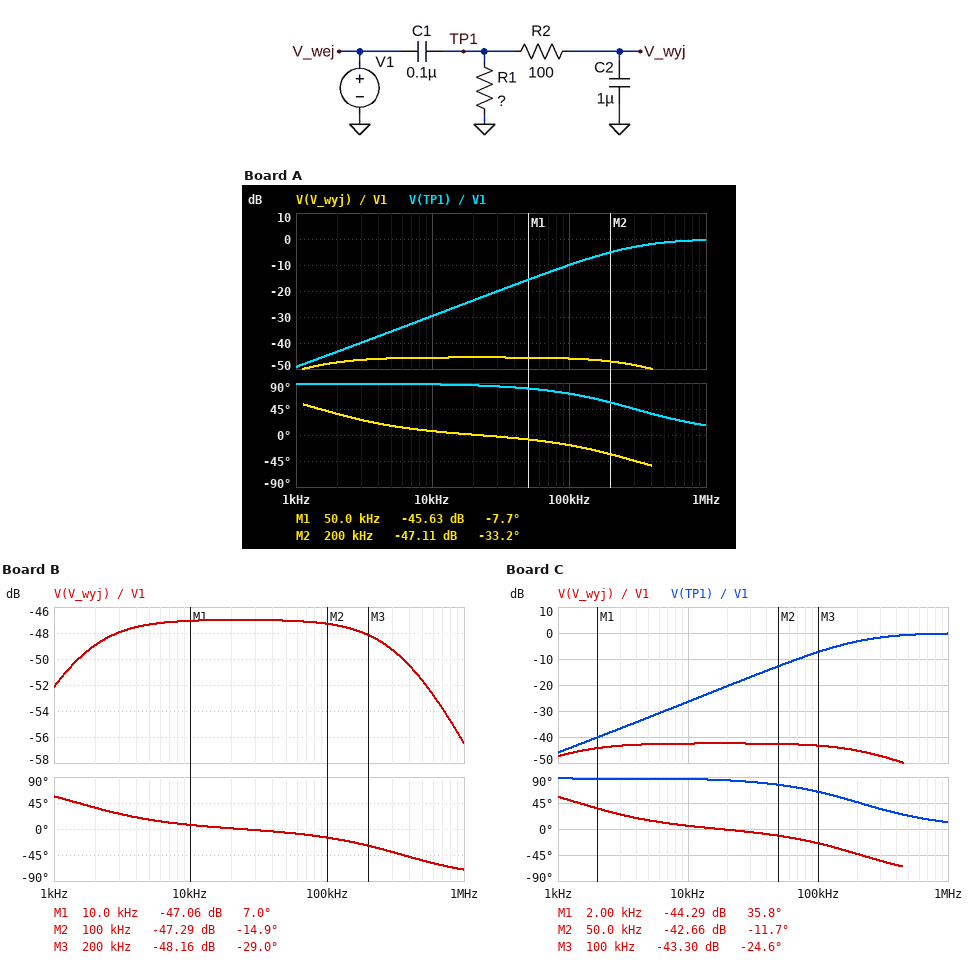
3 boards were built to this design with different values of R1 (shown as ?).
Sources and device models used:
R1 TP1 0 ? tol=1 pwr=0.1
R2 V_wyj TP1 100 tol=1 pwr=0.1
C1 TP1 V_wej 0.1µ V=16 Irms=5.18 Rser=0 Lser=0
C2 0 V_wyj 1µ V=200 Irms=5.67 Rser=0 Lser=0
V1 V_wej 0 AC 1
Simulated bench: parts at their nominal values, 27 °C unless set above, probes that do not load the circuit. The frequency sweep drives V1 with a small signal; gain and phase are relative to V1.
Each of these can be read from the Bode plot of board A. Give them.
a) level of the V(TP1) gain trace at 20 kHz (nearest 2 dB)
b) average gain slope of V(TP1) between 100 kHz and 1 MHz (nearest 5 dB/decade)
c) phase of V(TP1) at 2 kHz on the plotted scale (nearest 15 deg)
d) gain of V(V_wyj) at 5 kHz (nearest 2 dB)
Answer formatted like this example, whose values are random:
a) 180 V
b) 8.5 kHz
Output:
a) -24 dB
b) 10 dB/decade
c) 90 deg
d) -46 dB
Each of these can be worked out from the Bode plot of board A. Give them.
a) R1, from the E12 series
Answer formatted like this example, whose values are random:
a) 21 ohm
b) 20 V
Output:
a) 5.6 Ω
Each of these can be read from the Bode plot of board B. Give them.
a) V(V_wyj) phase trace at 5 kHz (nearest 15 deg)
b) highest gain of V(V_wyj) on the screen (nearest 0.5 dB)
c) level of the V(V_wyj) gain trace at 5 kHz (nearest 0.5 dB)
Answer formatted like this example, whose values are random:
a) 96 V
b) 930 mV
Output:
a) 15 deg
b) -47.0 dB
c) -47.5 dB
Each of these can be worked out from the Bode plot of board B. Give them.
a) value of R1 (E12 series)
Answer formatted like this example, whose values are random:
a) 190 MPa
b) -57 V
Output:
a) 4.7 Ω
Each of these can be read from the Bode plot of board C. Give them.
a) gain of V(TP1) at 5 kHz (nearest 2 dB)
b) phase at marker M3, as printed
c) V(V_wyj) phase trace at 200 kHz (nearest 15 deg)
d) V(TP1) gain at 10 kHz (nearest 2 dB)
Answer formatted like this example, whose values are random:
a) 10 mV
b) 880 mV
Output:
a) -32 dB
b) -24.6 deg
c) -45 deg
d) -26 dB
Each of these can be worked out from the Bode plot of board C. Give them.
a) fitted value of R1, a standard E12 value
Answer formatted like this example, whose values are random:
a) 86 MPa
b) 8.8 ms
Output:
a) 8.2 Ω
